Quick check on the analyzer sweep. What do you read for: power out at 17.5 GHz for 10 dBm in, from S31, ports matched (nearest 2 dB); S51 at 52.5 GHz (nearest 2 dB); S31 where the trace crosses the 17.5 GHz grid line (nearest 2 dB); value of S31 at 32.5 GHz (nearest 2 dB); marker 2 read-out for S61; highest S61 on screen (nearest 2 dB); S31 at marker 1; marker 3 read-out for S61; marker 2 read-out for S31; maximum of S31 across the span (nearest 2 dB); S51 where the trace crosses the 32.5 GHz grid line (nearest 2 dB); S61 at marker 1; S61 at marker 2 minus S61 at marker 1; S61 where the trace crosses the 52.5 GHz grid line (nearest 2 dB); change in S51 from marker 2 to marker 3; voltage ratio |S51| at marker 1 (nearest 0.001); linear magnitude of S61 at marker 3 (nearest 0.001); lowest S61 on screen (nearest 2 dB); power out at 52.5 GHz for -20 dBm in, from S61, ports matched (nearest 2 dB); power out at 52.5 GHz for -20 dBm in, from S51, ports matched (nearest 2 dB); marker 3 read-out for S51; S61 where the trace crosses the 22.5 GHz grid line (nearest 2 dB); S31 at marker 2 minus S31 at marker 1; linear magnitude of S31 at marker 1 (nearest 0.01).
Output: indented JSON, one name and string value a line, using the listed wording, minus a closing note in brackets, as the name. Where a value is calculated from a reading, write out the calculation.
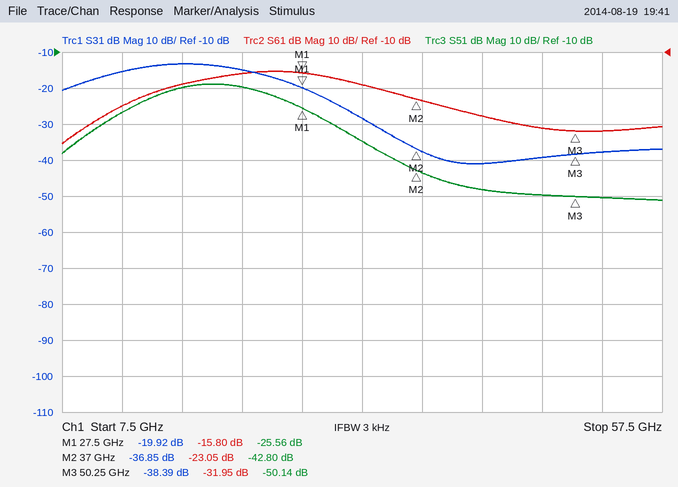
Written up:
{
  "power out at 17.5 GHz for 10 dBm in, from S31, ports matched": "10 dBm + (-14 dB) = -4 dBm",
  "S51 at 52.5 GHz": "-50 dB",
  "S31 where the trace crosses the 17.5 GHz grid line": "-14 dB",
  "value of S31 at 32.5 GHz": "-28 dB",
  "marker 2 read-out for S61": "-23.05 dB",
  "highest S61 on screen": "-16 dB",
  "S31 at marker 1": "-19.92 dB",
  "marker 3 read-out for S61": "-31.95 dB",
  "marker 2 read-out for S31": "-36.85 dB",
  "maximum of S31 across the span": "-14 dB",
  "S51 where the trace crosses the 32.5 GHz grid line": "-34 dB",
  "S61 at marker 1": "-15.80 dB",
  "S61 at marker 2 minus S61 at marker 1": "-23.05 − (-15.8) = -7.25 dB",
  "S61 where the trace crosses the 52.5 GHz grid line": "-32 dB",
  "change in S51 from marker 2 to marker 3": "-50.14 − (-42.8) = -7.34 dB",
  "voltage ratio |S51| at marker 1": "10^(-25.56/20) ≈ 0.053",
  "linear magnitude of S61 at marker 3": "10^(-31.95/20) ≈ 0.025",
  "lowest S61 on screen": "-36 dB",
  "power out at 52.5 GHz for -20 dBm in, from S61, ports matched": "-20 dBm + (-32 dB) = -52 dBm",
  "power out at 52.5 GHz for -20 dBm in, from S51, ports matched": "-20 dBm + (-50 dB) = -70 dBm",
  "marker 3 read-out for S51": "-50.14 dB",
  "S61 where the trace crosses the 22.5 GHz grid line": "-16 dB",
  "S31 at marker 2 minus S31 at marker 1": "-36.85 − (-19.92) = -16.93 dB",
  "linear magnitude of S31 at marker 1": "10^(-19.92/20) ≈ 0.10"
}
